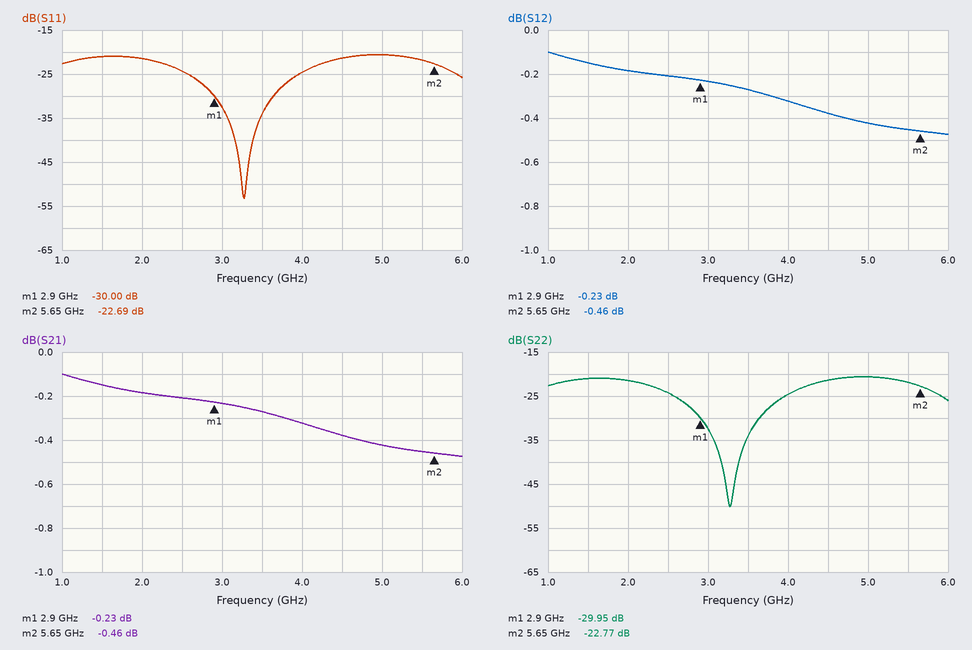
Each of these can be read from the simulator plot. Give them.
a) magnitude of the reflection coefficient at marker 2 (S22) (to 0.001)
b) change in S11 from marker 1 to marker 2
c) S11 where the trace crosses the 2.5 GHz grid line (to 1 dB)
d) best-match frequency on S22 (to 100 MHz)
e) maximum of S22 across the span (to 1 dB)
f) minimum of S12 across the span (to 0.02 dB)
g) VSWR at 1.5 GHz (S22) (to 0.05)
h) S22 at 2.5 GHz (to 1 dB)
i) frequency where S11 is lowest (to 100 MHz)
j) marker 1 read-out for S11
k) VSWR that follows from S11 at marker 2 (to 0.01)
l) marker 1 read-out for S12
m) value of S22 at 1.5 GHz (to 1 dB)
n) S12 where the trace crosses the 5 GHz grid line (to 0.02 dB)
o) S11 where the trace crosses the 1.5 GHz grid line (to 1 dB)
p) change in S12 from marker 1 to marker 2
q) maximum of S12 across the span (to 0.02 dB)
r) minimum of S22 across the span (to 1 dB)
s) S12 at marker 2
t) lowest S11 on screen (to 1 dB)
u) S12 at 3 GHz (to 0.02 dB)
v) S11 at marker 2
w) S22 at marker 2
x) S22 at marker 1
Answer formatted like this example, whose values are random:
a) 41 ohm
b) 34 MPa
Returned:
a) 0.073
b) 7.31 dB
c) -24 dB
d) 3.3 GHz
e) -21 dB
f) -0.48 dB
g) 1.20
h) -24 dB
i) 3.3 GHz
j) -30.00 dB
k) 1.16
l) -0.23 dB
m) -21 dB
n) -0.42 dB
o) -21 dB
p) -0.23 dB
q) -0.10 dB
r) -50 dB
s) -0.46 dB
t) -53 dB
u) -0.24 dB
v) -22.69 dB
w) -22.77 dB
x) -29.95 dB
